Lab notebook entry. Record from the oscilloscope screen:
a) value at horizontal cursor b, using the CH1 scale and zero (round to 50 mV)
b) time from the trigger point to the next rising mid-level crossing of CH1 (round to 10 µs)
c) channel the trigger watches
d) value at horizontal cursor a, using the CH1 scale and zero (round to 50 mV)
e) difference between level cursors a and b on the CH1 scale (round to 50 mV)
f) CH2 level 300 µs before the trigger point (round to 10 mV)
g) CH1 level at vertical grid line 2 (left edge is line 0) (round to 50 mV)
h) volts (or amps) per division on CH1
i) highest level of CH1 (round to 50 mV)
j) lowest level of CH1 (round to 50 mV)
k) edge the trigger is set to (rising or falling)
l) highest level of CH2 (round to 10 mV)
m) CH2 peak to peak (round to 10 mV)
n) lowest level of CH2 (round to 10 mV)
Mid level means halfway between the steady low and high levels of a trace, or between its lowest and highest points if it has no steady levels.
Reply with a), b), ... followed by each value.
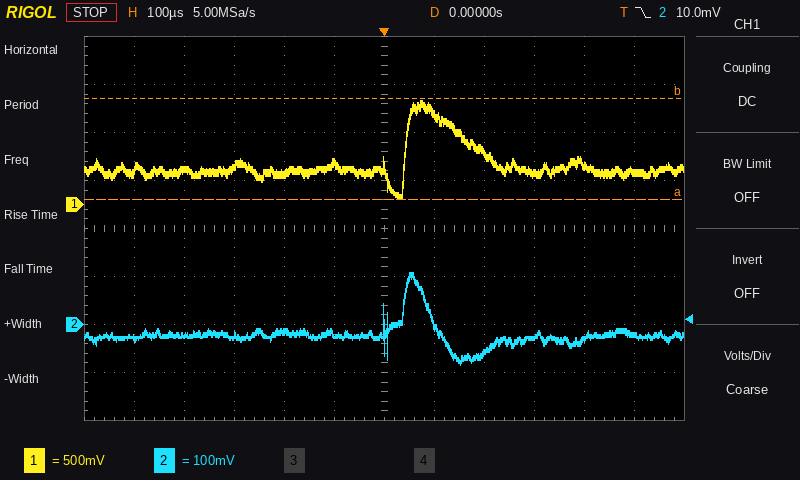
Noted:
a) 1.10 V
b) 40 µs
c) CH2
d) 50 mV
e) 1.05 V
f) -20 mV
g) 350 mV
h) 500 mV
i) 1.10 V
j) 50 mV
k) falling
l) 110 mV
m) 190 mV
n) -80 mV
